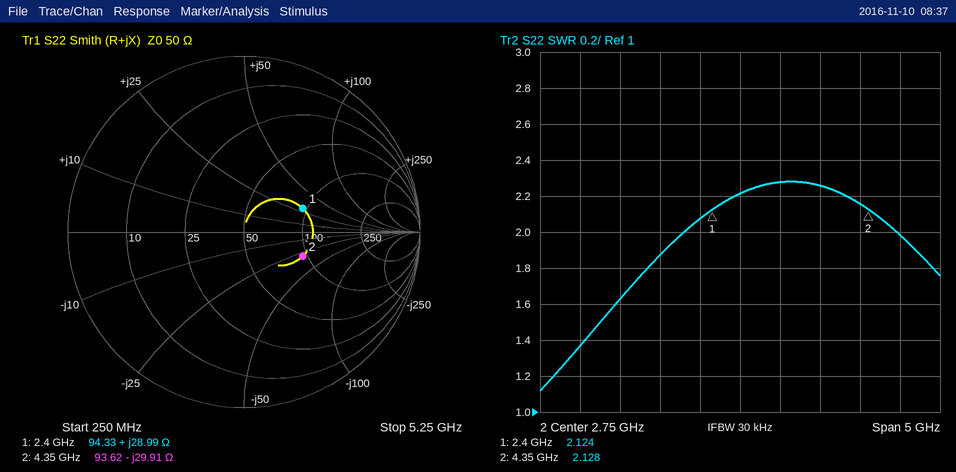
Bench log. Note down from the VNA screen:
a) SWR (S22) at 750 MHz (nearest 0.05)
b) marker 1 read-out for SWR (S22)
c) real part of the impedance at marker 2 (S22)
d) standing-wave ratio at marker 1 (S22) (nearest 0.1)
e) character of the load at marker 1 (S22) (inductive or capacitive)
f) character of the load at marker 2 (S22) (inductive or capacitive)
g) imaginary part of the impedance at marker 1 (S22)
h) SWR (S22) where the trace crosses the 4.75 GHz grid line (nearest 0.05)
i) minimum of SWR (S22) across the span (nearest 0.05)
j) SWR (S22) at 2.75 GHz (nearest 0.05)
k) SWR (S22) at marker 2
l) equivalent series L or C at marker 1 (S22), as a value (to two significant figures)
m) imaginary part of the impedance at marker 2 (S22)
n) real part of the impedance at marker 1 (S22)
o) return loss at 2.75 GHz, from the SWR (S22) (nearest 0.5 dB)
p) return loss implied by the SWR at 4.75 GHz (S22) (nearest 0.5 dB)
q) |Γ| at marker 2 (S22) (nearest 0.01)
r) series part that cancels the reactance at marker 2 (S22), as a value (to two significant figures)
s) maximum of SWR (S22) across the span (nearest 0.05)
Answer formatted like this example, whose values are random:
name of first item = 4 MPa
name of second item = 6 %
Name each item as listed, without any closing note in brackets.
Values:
SWR (S22) at 750 MHz = 1.35
marker 1 read-out for SWR = 2.124
real part of the impedance at marker 2 = 93.62 Ω
standing-wave ratio at marker 1 (S22) = 2.1
character of the load at marker 1 (S22) = inductive
character of the load at marker 2 (S22) = capacitive
imaginary part of the impedance at marker 1 = +28.99 Ω
SWR (S22) where the trace crosses the 4.75 GHz grid line = 2.00
minimum of SWR (S22) across the span = 1.10
SWR (S22) at 2.75 GHz = 2.20
SWR (S22) at marker 2 = 2.128
equivalent series L or C at marker 1 (S22), as a value = 1.9 nH
imaginary part of the impedance at marker 2 = -29.91 Ω
real part of the impedance at marker 1 = 94.33 Ω
return loss at 2.75 GHz, from the SWR (S22) = 8.5 dB
return loss implied by the SWR at 4.75 GHz (S22) = 9.5 dB
|Γ| at marker 2 (S22) = 0.36
series part that cancels the reactance at marker 2 (S22), as a value = 1.1 nH
maximum of SWR (S22) across the span = 2.30
